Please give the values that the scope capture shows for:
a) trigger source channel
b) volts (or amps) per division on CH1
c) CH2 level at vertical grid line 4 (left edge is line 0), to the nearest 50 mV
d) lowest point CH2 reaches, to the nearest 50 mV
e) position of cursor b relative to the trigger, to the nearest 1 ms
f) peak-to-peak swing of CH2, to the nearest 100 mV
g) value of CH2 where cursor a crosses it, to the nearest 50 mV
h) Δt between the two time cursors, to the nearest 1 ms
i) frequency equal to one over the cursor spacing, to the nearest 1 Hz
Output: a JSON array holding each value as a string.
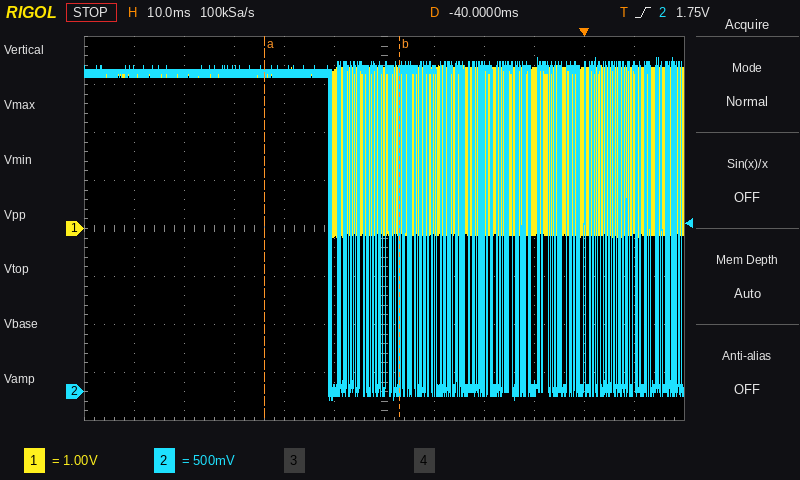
["CH2", "1 V", "3.30 V", "-100 mV", "-37 ms", "3.60 V", "3.30 V", "27 ms", "37 Hz"]
